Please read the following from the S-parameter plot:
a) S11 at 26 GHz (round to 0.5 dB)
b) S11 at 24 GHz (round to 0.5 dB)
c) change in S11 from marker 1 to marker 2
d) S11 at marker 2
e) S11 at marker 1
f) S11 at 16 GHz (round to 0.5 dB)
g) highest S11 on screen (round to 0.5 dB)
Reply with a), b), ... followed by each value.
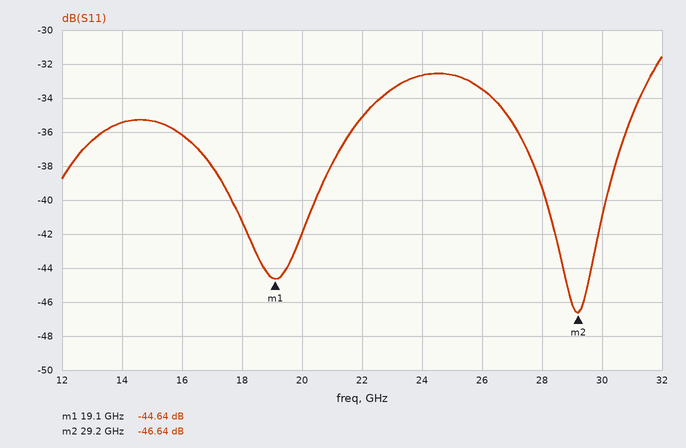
a) -33.5 dB
b) -32.5 dB
c) -2.00 dB
d) -46.64 dB
e) -44.64 dB
f) -36.0 dB
g) -31.5 dB
